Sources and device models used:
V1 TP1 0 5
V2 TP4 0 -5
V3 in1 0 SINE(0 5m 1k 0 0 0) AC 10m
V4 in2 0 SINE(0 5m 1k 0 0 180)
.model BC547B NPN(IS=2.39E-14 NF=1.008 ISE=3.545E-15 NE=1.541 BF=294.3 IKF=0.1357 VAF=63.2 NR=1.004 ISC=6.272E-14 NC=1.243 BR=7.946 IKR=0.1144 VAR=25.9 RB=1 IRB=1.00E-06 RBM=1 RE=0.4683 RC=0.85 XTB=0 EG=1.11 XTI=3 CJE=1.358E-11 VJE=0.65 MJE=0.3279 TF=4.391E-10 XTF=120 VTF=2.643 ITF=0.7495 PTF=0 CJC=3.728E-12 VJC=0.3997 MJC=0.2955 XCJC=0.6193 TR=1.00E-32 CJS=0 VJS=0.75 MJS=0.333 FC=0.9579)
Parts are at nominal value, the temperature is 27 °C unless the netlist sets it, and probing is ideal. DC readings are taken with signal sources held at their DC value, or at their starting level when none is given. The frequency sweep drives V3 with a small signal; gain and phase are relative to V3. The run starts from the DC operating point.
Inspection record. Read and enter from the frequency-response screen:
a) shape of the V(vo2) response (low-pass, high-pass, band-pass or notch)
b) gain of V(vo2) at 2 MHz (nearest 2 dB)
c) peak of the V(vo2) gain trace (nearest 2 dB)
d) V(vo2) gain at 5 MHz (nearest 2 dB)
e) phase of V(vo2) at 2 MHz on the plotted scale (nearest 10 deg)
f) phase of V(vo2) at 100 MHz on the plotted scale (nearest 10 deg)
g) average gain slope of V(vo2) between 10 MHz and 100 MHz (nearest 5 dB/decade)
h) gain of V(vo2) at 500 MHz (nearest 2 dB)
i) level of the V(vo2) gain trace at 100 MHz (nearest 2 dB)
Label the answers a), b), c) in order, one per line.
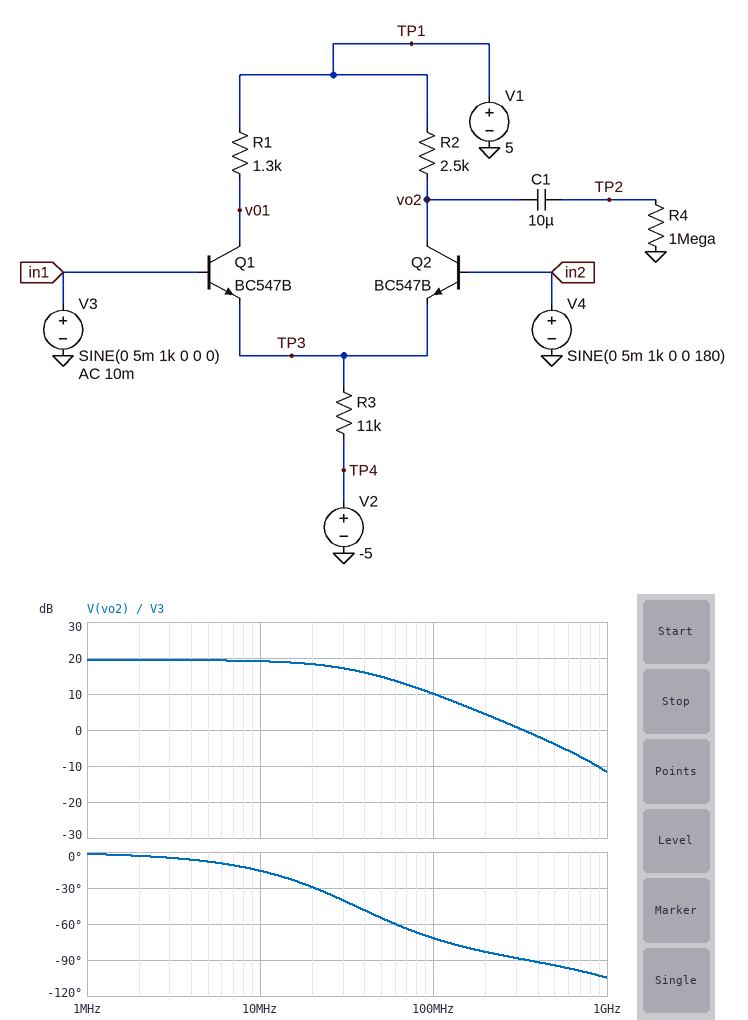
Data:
a) low-pass
b) 20 dB
c) 20 dB
d) 20 dB
e) 0 deg
f) -70 deg
g) -10 dB/decade
h) -4 dB
i) 10 dB
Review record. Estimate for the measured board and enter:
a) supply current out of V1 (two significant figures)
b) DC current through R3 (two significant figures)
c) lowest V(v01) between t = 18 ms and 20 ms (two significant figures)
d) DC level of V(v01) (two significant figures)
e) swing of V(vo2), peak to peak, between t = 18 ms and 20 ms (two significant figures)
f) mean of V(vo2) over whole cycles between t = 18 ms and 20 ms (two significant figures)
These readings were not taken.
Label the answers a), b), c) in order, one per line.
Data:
a) 400 µA
b) 400 µA
c) 4.7 V
d) 4.7 V
e) 190 mV
f) 4.5 V
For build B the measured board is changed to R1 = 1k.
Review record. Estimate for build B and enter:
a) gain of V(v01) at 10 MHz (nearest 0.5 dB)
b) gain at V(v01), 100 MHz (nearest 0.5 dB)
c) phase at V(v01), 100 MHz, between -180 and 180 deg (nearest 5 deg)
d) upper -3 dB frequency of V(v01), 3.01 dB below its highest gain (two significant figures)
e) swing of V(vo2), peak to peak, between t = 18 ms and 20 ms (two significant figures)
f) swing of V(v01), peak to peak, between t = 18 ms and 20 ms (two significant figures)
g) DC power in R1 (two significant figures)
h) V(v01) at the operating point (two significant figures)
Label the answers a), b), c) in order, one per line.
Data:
a) 11.5 dB
b) 8.5 dB
c) 115 deg
d) 99 MHz
e) 190 mV
f) 75 mV
g) 40 µW
h) 4.8 V
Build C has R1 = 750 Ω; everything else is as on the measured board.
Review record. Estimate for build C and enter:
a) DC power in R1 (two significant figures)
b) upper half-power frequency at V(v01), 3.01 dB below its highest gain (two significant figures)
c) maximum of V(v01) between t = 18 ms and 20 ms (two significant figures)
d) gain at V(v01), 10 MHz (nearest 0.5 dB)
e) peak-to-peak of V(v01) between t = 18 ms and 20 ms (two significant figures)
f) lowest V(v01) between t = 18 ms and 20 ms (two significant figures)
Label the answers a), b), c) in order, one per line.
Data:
a) 30 µW
b) 140 MHz
c) 4.9 V
d) 9.0 dB
e) 56 mV
f) 4.8 V
